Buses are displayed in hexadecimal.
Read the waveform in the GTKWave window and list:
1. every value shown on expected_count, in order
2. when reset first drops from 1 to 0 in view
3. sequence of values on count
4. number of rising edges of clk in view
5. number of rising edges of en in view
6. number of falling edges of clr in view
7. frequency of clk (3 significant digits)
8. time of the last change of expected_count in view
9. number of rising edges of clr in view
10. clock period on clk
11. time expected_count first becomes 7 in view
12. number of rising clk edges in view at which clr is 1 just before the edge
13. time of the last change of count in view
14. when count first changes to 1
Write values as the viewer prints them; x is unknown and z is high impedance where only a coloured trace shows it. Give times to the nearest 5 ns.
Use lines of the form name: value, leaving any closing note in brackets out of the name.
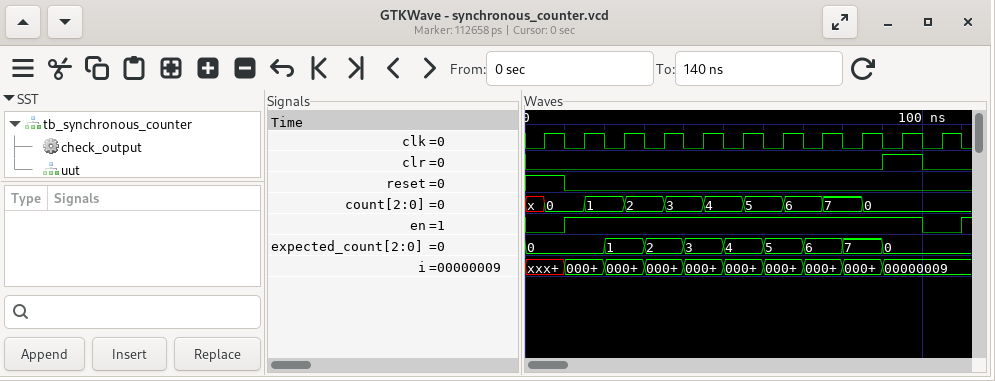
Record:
every value shown on expected_count, in order: 0, 1, 2, 3, 4, 5, 6, 7, 0
when reset first drops from 1 to 0 in view: 10 ns
sequence of values on count: x, 0, 1, 2, 3, 4, 5, 6, 7, 0
number of rising edges of clk in view: 11
number of rising edges of en in view: 2
number of falling edges of clr in view: 1
frequency of clk: 100 MHz
time of the last change of expected_count in view: 90 ns
number of rising edges of clr in view: 1
clock period on clk: 10 ns
time expected_count first becomes 7 in view: 80 ns
number of rising clk edges in view at which clr is 1 just before the edge: 1
time of the last change of count in view: 85 ns
when count first changes to 1: 15 ns
